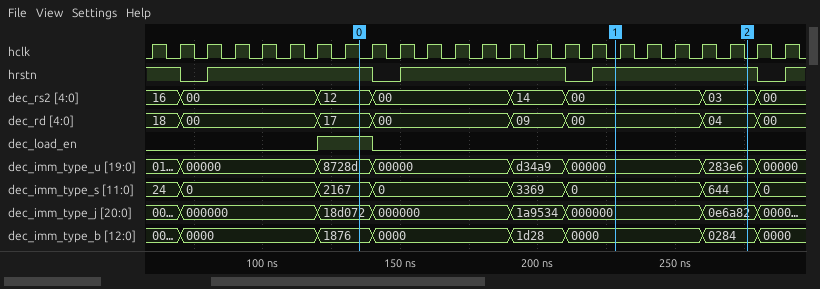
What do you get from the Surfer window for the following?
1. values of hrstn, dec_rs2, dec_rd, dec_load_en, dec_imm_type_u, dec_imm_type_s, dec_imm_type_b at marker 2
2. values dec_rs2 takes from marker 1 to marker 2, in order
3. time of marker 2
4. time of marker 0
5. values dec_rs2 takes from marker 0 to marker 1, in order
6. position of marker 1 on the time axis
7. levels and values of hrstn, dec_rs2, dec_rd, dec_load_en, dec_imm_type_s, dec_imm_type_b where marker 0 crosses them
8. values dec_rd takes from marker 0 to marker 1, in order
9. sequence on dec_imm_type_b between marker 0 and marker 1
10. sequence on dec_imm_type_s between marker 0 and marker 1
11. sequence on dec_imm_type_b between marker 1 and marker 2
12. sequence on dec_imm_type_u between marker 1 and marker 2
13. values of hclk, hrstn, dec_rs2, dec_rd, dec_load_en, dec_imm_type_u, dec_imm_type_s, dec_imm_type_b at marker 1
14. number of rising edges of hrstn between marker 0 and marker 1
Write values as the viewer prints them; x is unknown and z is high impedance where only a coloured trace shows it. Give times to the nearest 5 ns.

hrstn=1, dec_rs2=03, dec_rd=04, dec_load_en=0, dec_imm_type_u=283e6, dec_imm_type_s=644, dec_imm_type_b=0284
00, 03
275 ns
135 ns
12, 00, 14, 00
230 ns
hrstn=1, dec_rs2=12, dec_rd=17, dec_load_en=1, dec_imm_type_s=2167, dec_imm_type_b=1876
17, 00, 09, 00
1876, 0000, 1d28, 0000
2167, 0, 3369, 0
0000, 0284
00000, 283e6
hclk=0, hrstn=1, dec_rs2=00, dec_rd=00, dec_load_en=0, dec_imm_type_u=00000, dec_imm_type_s=0, dec_imm_type_b=0000
2
